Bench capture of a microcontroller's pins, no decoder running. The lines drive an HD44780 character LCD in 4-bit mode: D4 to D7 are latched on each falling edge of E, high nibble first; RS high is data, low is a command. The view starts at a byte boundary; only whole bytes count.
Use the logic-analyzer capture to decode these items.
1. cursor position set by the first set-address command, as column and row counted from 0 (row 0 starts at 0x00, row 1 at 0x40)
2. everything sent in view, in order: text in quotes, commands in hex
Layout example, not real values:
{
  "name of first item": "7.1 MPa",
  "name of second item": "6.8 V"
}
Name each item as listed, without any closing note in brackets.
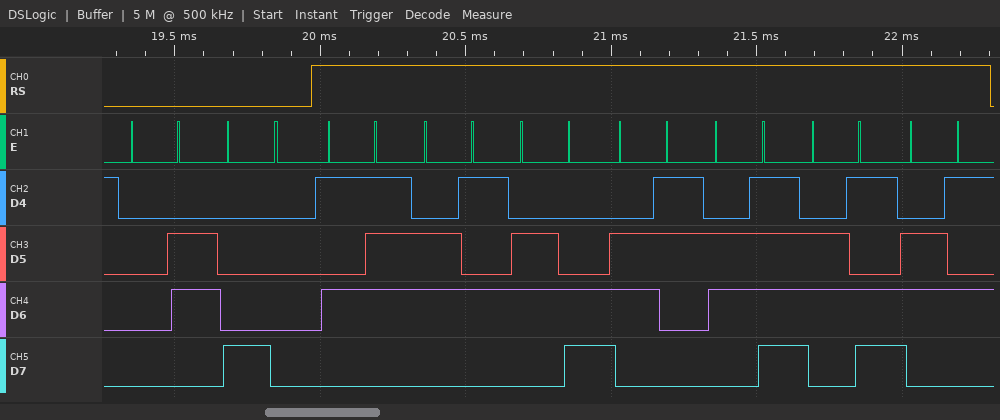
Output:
{
  "cursor position set by the first set-address command, as column and row counted from 0": "column 0, row 0",
  "everything sent in view, in order: text in quotes, commands in hex": "0x06 0x80 \"Welcome\""
}
